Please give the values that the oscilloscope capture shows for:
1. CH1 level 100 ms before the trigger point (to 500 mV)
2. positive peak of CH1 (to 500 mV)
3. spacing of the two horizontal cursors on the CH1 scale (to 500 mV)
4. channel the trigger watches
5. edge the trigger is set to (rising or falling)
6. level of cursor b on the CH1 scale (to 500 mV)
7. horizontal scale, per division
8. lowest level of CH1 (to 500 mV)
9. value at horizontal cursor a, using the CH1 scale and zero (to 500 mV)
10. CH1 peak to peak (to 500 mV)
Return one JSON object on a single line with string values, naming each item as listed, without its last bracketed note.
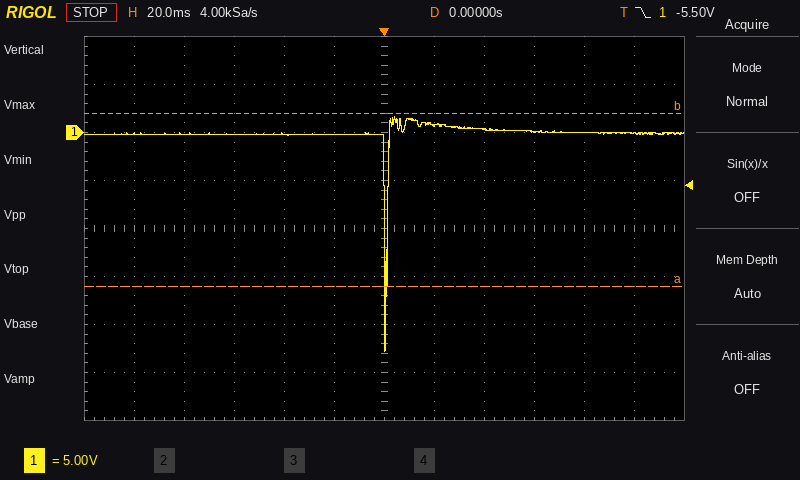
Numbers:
{"CH1 level 100 ms before the trigger point": "0.0 V", "positive peak of CH1": "1.5 V", "spacing of the two horizontal cursors on the CH1 scale": "18.0 V", "channel the trigger watches": "CH1", "edge the trigger is set to": "falling", "level of cursor b on the CH1 scale": "2.0 V", "horizontal scale, per division": "20 ms", "lowest level of CH1": "-23.0 V", "value at horizontal cursor a, using the CH1 scale and zero": "-16.0 V", "CH1 peak to peak": "24.5 V"}
